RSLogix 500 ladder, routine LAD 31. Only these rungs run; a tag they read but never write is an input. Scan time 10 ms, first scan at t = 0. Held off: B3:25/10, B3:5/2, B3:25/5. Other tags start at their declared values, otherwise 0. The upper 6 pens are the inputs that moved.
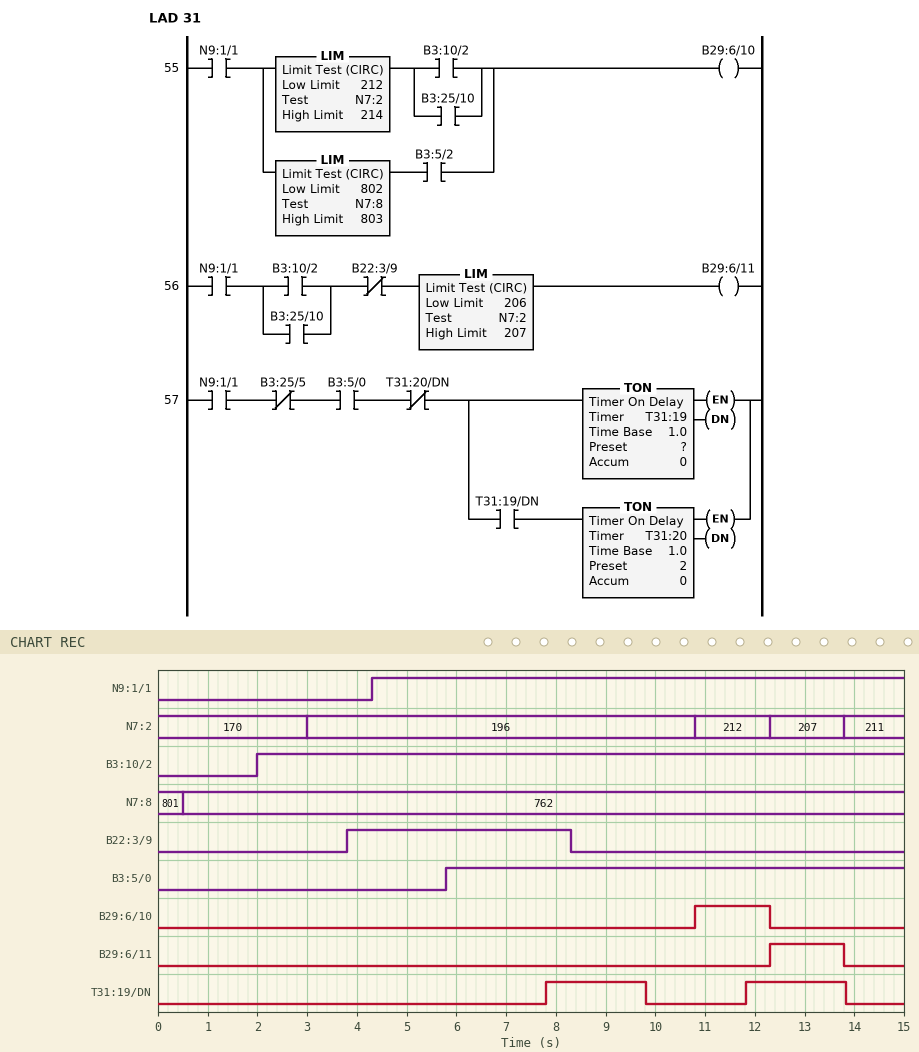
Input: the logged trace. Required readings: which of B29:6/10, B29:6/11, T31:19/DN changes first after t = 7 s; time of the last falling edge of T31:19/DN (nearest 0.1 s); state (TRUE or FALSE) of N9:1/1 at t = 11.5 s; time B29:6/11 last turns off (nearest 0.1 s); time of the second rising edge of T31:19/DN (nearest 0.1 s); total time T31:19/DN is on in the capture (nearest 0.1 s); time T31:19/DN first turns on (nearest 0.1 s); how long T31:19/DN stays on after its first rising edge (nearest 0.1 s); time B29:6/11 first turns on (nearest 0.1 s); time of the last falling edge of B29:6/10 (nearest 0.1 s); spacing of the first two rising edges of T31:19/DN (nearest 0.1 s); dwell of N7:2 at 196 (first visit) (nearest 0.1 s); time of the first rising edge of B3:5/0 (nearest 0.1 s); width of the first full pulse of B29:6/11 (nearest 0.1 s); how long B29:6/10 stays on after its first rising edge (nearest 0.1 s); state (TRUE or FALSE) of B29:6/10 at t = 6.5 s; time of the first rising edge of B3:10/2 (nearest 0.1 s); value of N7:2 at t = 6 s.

T31:19/DN
13.8 s
TRUE
13.8 s
11.8 s
4.0 s
7.8 s
2.0 s
12.3 s
12.3 s
4.0 s
7.8 s
5.8 s
1.5 s
1.5 s
FALSE
2.0 s
196
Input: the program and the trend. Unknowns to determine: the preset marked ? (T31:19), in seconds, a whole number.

2 s
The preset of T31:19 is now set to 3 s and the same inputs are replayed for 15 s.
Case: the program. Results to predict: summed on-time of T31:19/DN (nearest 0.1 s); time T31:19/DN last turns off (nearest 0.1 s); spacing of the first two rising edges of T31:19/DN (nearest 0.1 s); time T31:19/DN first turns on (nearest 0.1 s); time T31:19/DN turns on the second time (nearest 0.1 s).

3.2 s
10.8 s
5.0 s
8.8 s
13.8 s
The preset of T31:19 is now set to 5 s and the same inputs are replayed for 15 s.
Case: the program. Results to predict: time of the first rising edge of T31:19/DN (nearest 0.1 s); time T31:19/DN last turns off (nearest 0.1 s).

10.8 s
12.8 s
